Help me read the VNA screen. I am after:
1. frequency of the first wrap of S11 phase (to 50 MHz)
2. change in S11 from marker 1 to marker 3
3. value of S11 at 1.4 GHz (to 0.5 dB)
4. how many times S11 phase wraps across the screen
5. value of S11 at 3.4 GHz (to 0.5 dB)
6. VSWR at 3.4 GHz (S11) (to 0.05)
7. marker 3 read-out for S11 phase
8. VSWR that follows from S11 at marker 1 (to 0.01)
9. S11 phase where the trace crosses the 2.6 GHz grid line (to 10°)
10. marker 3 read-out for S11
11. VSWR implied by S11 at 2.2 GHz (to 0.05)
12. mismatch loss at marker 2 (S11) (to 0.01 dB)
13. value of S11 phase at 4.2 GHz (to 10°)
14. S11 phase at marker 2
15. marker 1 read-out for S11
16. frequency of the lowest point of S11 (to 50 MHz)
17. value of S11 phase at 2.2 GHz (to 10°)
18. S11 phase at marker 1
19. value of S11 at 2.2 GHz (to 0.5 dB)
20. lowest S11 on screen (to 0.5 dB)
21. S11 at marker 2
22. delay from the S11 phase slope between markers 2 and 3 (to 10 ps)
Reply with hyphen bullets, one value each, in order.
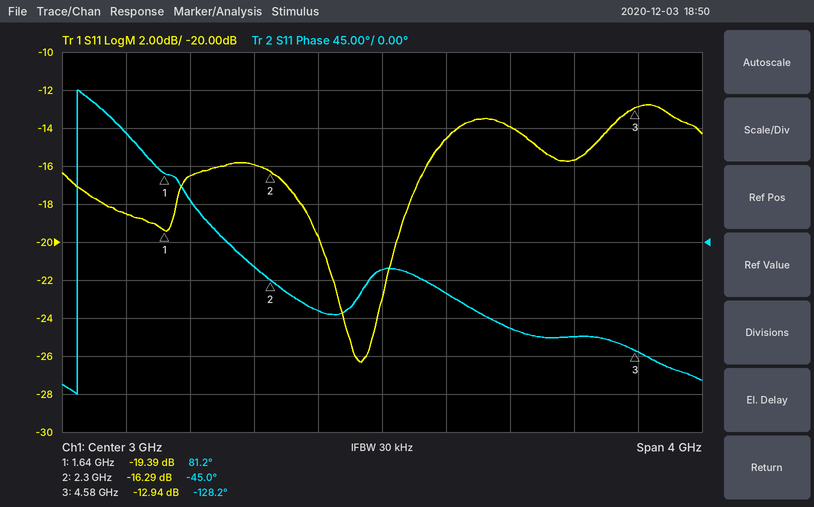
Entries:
- 1.10 GHz
- 6.45 dB
- -18.5 dB
- 1
- -14.5 dB
- 1.45
- -128.2°
- 1.24
- -80°
- -12.94 dB
- 1.40
- 0.10 dB
- -110°
- -45.0°
- -19.39 dB
- 2.85 GHz
- -30°
- 81.2°
- -16.0 dB
- -26.5 dB
- -16.29 dB
- 100 ps
